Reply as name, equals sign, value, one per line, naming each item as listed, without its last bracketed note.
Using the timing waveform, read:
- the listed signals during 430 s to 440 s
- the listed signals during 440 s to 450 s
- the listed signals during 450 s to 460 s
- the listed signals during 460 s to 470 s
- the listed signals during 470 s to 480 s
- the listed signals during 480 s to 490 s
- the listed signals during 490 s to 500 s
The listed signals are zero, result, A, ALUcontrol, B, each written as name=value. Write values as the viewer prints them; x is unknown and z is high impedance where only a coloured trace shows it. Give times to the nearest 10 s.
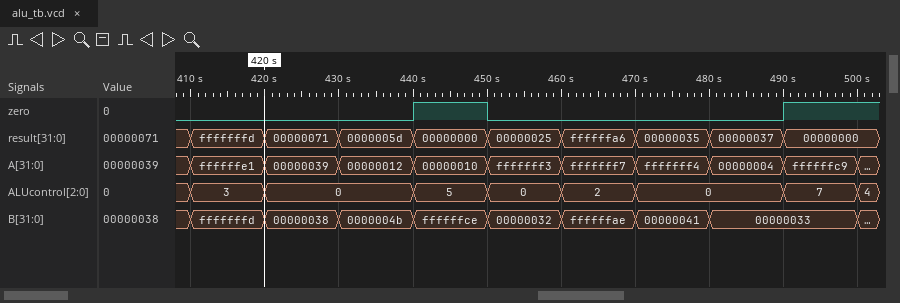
the listed signals during 430 s to 440 s = zero=0, result=0000005d, A=00000012, ALUcontrol=0, B=0000004b
the listed signals during 440 s to 450 s = zero=1, result=00000000, A=00000010, ALUcontrol=5, B=ffffffce
the listed signals during 450 s to 460 s = zero=0, result=00000025, A=fffffff3, ALUcontrol=0, B=00000032
the listed signals during 460 s to 470 s = zero=0, result=ffffffa6, A=fffffff7, ALUcontrol=2, B=ffffffae
the listed signals during 470 s to 480 s = zero=0, result=00000035, A=fffffff4, ALUcontrol=0, B=00000041
the listed signals during 480 s to 490 s = zero=0, result=00000037, A=00000004, ALUcontrol=0, B=00000033
the listed signals during 490 s to 500 s = zero=1, result=00000000, A=ffffffc9, ALUcontrol=7, B=00000033
